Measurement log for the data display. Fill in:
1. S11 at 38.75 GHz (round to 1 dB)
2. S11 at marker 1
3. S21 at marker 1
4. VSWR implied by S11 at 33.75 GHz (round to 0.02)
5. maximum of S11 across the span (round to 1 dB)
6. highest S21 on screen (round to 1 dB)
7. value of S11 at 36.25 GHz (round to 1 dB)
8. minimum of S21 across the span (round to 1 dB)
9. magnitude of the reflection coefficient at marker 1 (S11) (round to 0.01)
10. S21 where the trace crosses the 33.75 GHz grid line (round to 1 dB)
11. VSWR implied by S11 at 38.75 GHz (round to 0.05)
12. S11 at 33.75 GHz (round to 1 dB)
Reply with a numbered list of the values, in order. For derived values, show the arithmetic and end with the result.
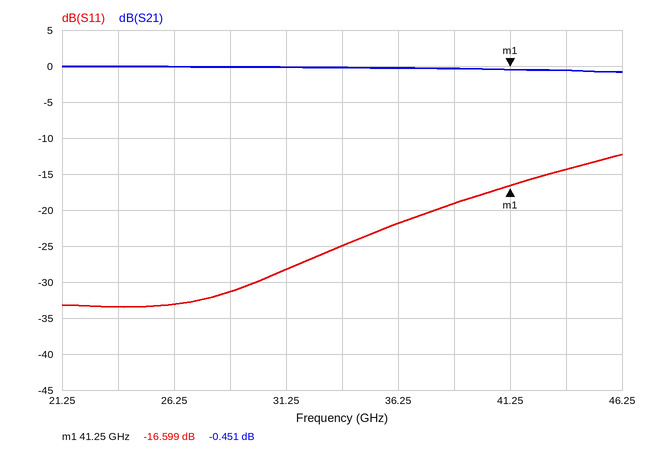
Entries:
1. -19 dB
2. -16.599 dB
3. -0.451 dB
4. |Γ| = 10^(-25/20) = 0.0562; VSWR = (1 + 0.0562)/(1 − 0.0562) ≈ 1.12
5. -12 dB
6. 0 dB
7. -22 dB
8. -1 dB
9. 10^(-16.599/20) ≈ 0.15
10. 0 dB
11. |Γ| = 10^(-19/20) = 0.1122; VSWR = (1 + 0.1122)/(1 − 0.1122) ≈ 1.25
12. -25 dB
